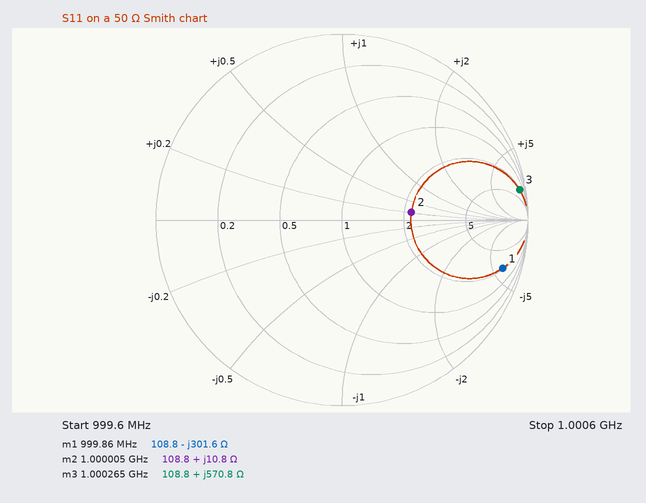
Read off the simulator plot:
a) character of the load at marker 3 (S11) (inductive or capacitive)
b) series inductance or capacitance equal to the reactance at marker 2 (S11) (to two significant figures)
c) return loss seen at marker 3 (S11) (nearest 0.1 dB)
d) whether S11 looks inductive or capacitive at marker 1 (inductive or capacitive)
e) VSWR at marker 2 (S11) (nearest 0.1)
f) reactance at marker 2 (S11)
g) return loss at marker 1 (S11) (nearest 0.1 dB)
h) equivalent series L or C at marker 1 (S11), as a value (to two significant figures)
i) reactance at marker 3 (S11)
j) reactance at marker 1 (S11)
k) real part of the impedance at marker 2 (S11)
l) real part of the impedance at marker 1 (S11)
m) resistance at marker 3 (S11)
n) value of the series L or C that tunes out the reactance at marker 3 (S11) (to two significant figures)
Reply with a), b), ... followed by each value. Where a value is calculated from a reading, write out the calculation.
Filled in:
a) inductive
b) L = 10.8 Ω/(2π × 1.000005 GHz) ≈ 1.7 nH
c) 0.3 dB
d) capacitive
e) 2.2
f) +10.8 Ω
g) 0.9 dB
h) C = 1/(2π × 999.86 MHz × 301.6 Ω) ≈ 528 fF, so 530 fF to two significant figures
i) +570.8 Ω
j) -301.6 Ω
k) 108.8 Ω
l) 108.8 Ω
m) 108.8 Ω
n) C = 1/(2π × 1.000265 GHz × 570.8 Ω) ≈ 279 fF, so 280 fF to two significant figures
